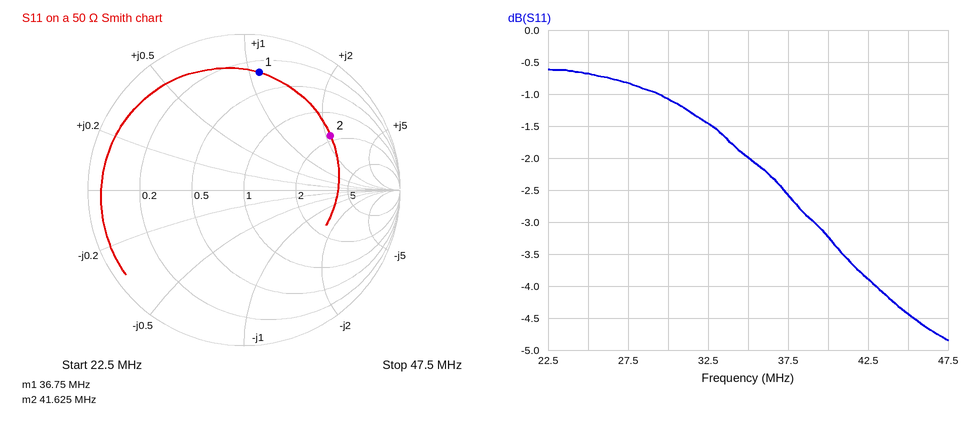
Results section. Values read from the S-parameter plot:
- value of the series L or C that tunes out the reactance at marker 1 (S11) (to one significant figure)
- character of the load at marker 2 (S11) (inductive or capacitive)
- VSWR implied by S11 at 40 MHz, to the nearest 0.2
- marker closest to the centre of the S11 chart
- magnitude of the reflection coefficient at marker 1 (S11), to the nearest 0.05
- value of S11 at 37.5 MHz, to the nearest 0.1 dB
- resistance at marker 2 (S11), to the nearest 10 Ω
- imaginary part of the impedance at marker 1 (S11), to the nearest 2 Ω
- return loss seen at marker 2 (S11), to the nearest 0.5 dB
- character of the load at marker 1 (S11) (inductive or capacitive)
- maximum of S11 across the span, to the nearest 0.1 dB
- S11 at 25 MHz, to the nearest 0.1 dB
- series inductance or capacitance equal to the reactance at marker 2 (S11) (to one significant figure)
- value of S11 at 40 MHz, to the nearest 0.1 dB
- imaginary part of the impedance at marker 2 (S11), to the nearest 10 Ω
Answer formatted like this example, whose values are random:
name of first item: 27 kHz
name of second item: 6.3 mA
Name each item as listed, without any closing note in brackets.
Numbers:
value of the series L or C that tunes out the reactance at marker 1 (S11): 80 pF
character of the load at marker 2 (S11): inductive
VSWR implied by S11 at 40 MHz, to the nearest 0.2: 5.4
marker closest to the centre of the S11 chart: marker 2
magnitude of the reflection coefficient at marker 1 (S11), to the nearest 0.05: 0.75
value of S11 at 37.5 MHz, to the nearest 0.1 dB: -2.6 dB
resistance at marker 2 (S11), to the nearest 10 Ω: 90 Ω
imaginary part of the impedance at marker 1 (S11), to the nearest 2 Ω: +54 Ω
return loss seen at marker 2 (S11), to the nearest 0.5 dB: 3.5 dB
character of the load at marker 1 (S11): inductive
maximum of S11 across the span, to the nearest 0.1 dB: -0.6 dB
S11 at 25 MHz, to the nearest 0.1 dB: -0.7 dB
series inductance or capacitance equal to the reactance at marker 2 (S11): 400 nH
value of S11 at 40 MHz, to the nearest 0.1 dB: -3.2 dB
imaginary part of the impedance at marker 2 (S11), to the nearest 10 Ω: +110 Ω
